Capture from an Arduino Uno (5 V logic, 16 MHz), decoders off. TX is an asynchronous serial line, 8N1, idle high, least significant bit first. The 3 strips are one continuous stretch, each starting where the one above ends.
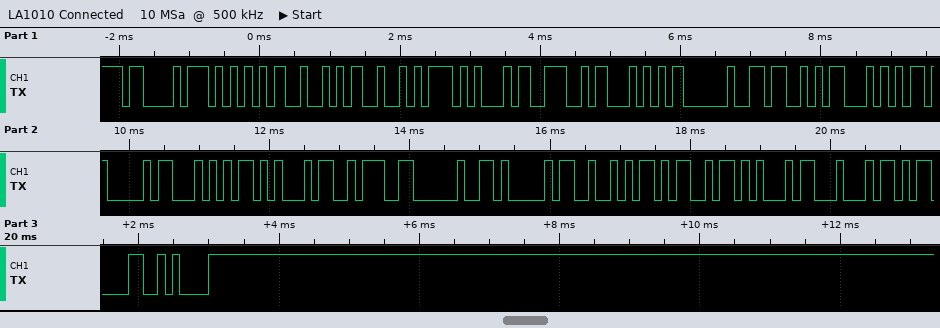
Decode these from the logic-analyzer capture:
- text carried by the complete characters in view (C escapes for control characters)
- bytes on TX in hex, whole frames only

"CURRENT STATE: ARMED\r\n"
43 55 52 52 45 4E 54 20 53 54 41 54 45 3A 20 41 52 4D 45 44 0D 0A
